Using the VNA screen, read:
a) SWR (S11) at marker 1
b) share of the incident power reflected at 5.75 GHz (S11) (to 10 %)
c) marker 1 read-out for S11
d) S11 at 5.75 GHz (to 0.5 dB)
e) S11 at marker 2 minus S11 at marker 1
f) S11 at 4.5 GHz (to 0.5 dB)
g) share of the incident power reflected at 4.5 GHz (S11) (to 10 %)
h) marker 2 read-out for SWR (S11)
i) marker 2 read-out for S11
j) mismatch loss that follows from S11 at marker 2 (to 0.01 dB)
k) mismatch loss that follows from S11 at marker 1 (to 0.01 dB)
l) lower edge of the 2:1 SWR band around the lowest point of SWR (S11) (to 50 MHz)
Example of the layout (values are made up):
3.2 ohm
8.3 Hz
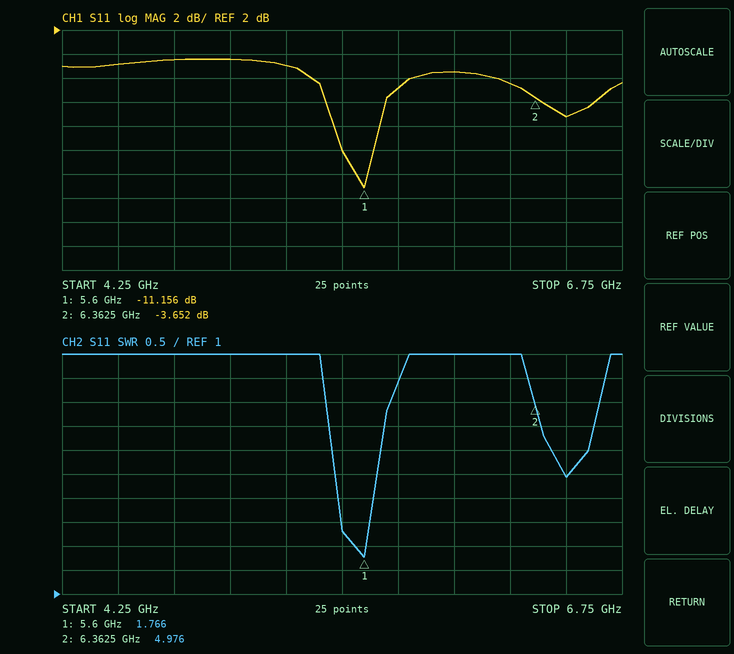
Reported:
1.766
50 %
-11.156 dB
-3.0 dB
7.504 dB
-1.0 dB
80 %
4.976
-3.652 dB
2.45 dB
0.35 dB
5.55 GHz
